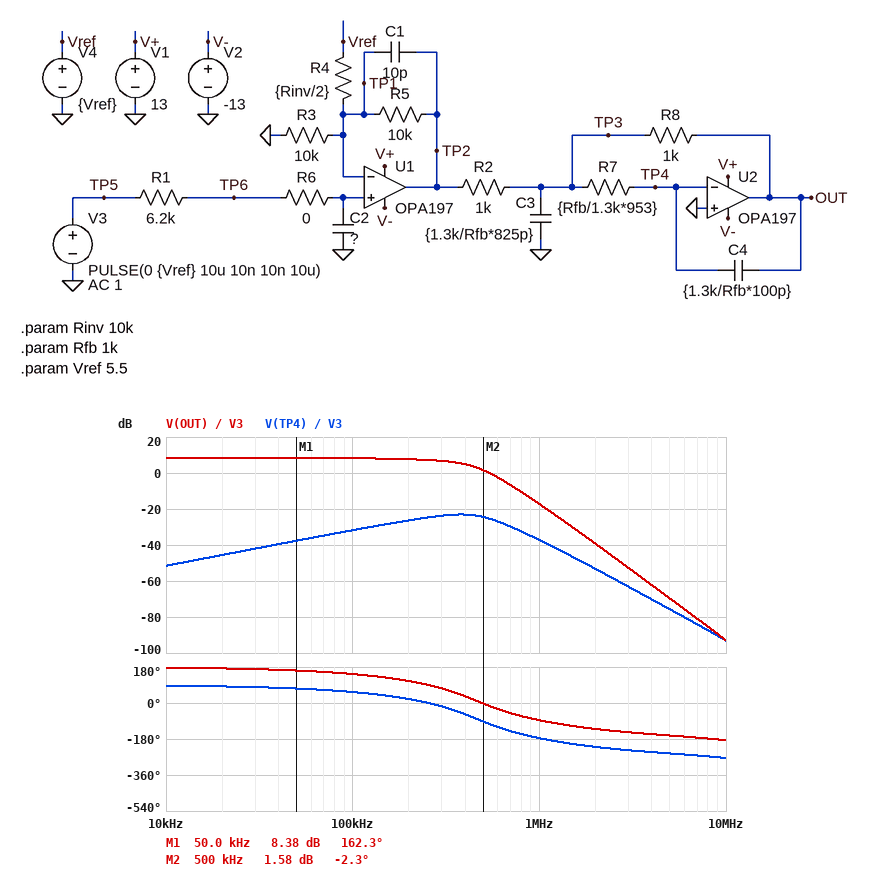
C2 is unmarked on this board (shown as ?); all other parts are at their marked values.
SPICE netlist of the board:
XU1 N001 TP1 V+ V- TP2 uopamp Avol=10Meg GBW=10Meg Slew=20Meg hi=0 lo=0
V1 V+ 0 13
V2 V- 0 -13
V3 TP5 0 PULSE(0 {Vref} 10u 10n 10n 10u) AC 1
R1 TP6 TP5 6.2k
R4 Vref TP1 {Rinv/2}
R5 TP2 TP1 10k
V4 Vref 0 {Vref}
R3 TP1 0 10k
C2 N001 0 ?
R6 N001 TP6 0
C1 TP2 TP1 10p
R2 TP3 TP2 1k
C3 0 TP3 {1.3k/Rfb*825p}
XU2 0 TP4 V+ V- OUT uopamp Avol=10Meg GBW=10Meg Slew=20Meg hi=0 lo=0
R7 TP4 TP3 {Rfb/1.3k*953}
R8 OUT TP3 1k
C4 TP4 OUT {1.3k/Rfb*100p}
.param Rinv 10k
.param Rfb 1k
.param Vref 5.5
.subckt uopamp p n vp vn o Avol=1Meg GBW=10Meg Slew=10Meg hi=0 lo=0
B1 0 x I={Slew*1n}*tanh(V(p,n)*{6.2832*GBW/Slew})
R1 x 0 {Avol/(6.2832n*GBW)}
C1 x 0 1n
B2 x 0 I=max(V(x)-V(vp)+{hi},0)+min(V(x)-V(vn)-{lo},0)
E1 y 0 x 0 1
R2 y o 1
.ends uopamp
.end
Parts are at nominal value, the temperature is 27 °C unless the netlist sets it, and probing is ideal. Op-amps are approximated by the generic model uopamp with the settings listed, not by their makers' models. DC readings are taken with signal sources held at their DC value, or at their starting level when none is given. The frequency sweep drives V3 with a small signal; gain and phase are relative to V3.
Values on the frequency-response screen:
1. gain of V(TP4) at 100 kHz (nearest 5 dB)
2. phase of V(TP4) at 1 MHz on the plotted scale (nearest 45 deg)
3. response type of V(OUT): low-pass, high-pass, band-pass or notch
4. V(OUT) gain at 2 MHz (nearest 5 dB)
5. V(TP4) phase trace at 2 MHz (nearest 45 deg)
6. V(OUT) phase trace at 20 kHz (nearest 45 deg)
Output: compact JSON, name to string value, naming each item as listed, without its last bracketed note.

{"gain of V(TP4) at 100 kHz": "-30 dB", "phase of V(TP4) at 1 MHz on the plotted scale": "-180 deg", "response type of V(OUT): low-pass, high-pass, band-pass or notch": "low-pass", "V(OUT) gain at 2 MHz": "-40 dB", "V(TP4) phase trace at 2 MHz": "-225 deg", "V(OUT) phase trace at 20 kHz": "180 deg"}
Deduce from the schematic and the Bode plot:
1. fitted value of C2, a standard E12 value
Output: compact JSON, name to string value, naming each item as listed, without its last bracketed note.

{"fitted value of C2, a standard E12 value": "120 pF"}
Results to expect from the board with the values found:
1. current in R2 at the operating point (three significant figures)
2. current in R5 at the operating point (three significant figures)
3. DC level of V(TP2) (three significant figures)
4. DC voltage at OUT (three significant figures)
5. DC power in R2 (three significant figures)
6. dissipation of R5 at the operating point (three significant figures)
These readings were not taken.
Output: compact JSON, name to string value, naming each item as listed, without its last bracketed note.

{"current in R2 at the operating point": "11.0 mA", "current in R5 at the operating point": "1.10 mA", "DC level of V(TP2)": "-11.0 V", "DC voltage at OUT": "11.0 V", "DC power in R2": "121 mW", "dissipation of R5 at the operating point": "12.1 mW"}
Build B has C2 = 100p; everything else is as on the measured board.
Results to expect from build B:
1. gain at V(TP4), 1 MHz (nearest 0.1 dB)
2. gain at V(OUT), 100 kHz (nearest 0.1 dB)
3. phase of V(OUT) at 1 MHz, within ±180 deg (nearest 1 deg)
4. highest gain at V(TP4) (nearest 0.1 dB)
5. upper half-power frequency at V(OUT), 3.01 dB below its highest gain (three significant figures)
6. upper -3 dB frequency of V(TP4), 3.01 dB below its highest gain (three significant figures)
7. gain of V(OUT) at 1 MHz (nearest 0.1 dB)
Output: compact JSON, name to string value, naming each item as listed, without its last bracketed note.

{"gain at V(TP4), 1 MHz": "-35.8 dB", "gain at V(OUT), 100 kHz": "8.3 dB", "phase of V(OUT) at 1 MHz, within ±180 deg": "-83 deg", "highest gain at V(TP4)": "-22.2 dB", "upper half-power frequency at V(OUT), 3.01 dB below its highest gain": "413 kHz", "upper -3 dB frequency of V(TP4), 3.01 dB below its highest gain": "577 kHz", "gain of V(OUT) at 1 MHz": "-15.8 dB"}
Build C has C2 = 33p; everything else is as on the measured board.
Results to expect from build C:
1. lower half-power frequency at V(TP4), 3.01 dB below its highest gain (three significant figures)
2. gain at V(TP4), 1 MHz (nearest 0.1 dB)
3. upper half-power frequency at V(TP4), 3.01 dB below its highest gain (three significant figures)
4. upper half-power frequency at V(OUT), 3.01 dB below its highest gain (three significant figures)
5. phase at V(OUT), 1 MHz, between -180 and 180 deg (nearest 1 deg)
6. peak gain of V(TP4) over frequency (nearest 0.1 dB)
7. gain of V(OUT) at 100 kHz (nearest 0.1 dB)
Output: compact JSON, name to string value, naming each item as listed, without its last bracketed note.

{"lower half-power frequency at V(TP4), 3.01 dB below its highest gain": "264 kHz", "gain at V(TP4), 1 MHz": "-29.4 dB", "upper half-power frequency at V(TP4), 3.01 dB below its highest gain": "646 kHz", "upper half-power frequency at V(OUT), 3.01 dB below its highest gain": "501 kHz", "phase at V(OUT), 1 MHz, between -180 and 180 deg": "-54 deg", "peak gain of V(TP4) over frequency": "-19.4 dB", "gain of V(OUT) at 100 kHz": "8.6 dB"}
